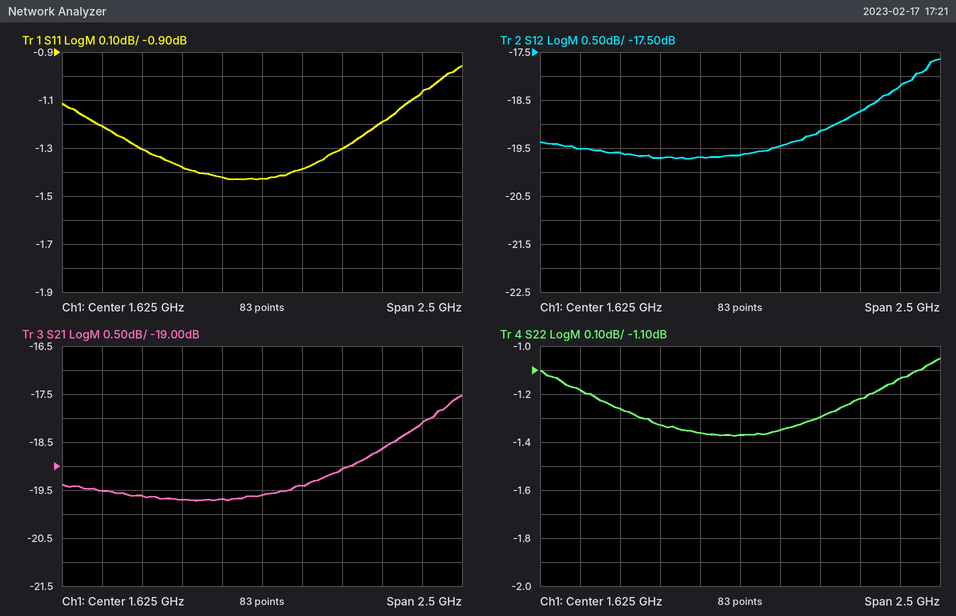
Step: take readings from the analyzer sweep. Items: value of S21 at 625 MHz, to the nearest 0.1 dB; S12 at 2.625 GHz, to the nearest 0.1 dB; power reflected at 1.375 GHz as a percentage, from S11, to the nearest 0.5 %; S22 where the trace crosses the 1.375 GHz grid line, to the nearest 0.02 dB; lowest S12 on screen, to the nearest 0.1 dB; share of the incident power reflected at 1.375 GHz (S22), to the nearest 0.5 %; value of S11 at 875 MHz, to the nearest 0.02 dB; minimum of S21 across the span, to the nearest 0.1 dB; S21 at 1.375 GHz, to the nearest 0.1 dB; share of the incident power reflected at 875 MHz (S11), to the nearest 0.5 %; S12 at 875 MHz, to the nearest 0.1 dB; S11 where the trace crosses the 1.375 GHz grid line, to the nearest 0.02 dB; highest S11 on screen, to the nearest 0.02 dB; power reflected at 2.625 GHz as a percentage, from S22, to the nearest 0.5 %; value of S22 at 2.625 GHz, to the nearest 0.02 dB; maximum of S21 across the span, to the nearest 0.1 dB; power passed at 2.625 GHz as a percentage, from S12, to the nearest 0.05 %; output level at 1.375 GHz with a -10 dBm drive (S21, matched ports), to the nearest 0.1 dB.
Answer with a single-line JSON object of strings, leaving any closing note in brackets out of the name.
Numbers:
{"value of S21 at 625 MHz, to the nearest 0.1 dB": "-19.5 dB", "S12 at 2.625 GHz, to the nearest 0.1 dB": "-18.2 dB", "power reflected at 1.375 GHz as a percentage, from S11, to the nearest 0.5 %": "72.0 %", "S22 where the trace crosses the 1.375 GHz grid line, to the nearest 0.02 dB": "-1.36 dB", "lowest S12 on screen, to the nearest 0.1 dB": "-19.7 dB", "share of the incident power reflected at 1.375 GHz (S22), to the nearest 0.5 %": "73.0 %", "value of S11 at 875 MHz, to the nearest 0.02 dB": "-1.30 dB", "minimum of S21 across the span, to the nearest 0.1 dB": "-19.7 dB", "S21 at 1.375 GHz, to the nearest 0.1 dB": "-19.7 dB", "share of the incident power reflected at 875 MHz (S11), to the nearest 0.5 %": "74.0 %", "S12 at 875 MHz, to the nearest 0.1 dB": "-19.6 dB", "S11 where the trace crosses the 1.375 GHz grid line, to the nearest 0.02 dB": "-1.42 dB", "highest S11 on screen, to the nearest 0.02 dB": "-0.96 dB", "power reflected at 2.625 GHz as a percentage, from S22, to the nearest 0.5 %": "77.0 %", "value of S22 at 2.625 GHz, to the nearest 0.02 dB": "-1.14 dB", "maximum of S21 across the span, to the nearest 0.1 dB": "-17.5 dB", "power passed at 2.625 GHz as a percentage, from S12, to the nearest 0.05 %": "1.50 %", "output level at 1.375 GHz with a -10 dBm drive (S21, matched ports), to the nearest 0.1 dB": "-29.7 dBm"}
